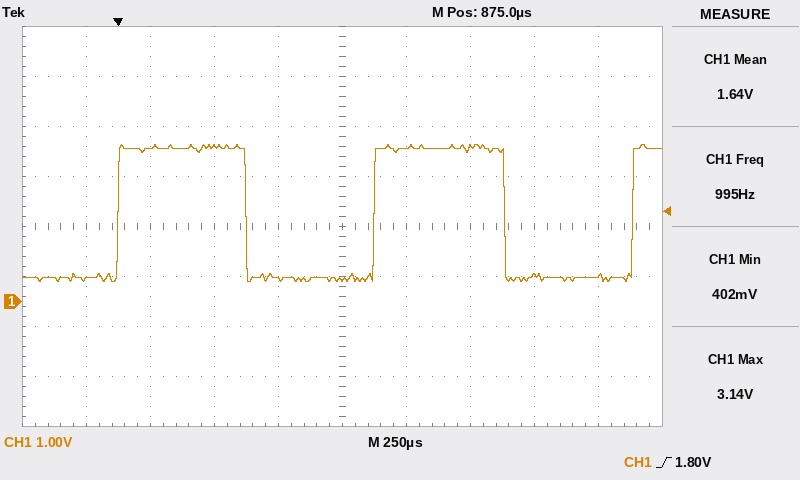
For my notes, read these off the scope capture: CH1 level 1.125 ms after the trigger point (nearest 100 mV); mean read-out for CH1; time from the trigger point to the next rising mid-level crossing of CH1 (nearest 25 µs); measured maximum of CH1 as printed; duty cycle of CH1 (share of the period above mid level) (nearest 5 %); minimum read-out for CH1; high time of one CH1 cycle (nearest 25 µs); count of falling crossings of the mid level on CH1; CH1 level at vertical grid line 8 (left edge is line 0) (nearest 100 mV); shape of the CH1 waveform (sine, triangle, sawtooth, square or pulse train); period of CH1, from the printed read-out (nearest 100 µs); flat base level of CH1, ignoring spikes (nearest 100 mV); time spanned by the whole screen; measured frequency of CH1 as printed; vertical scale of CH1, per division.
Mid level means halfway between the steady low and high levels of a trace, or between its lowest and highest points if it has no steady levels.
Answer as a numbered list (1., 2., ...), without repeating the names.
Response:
1. 3.1 V
2. 1.64 V
3. 1.000 ms
4. 3.14 V
5. 50 %
6. 402 mV
7. 500 µs
8. 2
9. 500 mV
10. square
11. 1.0 ms
12. 500 mV
13. 2.5 ms
14. 995 Hz
15. 1 V
